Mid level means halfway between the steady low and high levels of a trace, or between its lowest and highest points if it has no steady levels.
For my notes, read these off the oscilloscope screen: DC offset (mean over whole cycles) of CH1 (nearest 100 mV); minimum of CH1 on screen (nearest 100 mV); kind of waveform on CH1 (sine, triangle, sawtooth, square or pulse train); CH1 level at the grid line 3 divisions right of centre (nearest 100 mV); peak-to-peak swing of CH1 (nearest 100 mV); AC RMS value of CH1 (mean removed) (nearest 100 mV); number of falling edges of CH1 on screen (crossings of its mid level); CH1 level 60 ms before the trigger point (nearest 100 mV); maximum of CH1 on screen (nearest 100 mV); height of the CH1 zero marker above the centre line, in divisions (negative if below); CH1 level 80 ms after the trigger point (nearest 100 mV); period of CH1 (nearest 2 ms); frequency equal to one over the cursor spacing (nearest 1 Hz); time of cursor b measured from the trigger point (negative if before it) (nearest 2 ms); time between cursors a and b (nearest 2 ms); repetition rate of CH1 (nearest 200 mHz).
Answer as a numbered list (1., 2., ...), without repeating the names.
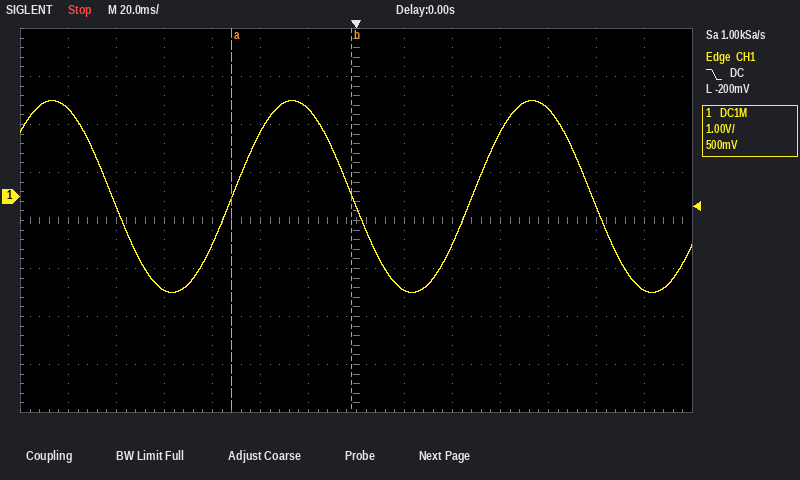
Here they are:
1. 0.0 V
2. -2.0 V
3. sine
4. 1.3 V
5. 4.0 V
6. 1.4 V
7. 3
8. -1.0 V
9. 2.0 V
10. +0.5 div
11. 1.8 V
12. 100 ms
13. 20 Hz
14. -2 ms
15. 50 ms
16. 10.0 Hz
